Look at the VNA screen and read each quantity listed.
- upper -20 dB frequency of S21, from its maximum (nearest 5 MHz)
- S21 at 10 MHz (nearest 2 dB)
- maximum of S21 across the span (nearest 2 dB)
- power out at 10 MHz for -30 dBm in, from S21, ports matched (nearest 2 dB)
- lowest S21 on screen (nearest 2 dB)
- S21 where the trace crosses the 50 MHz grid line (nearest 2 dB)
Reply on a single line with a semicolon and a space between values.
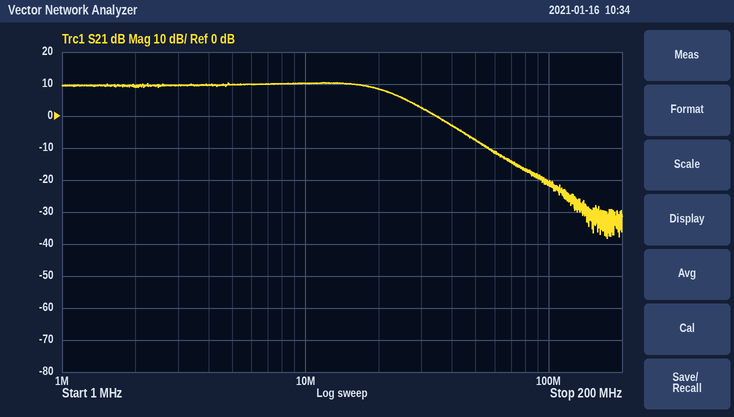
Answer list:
55 MHz; 10 dB; 10 dB; -20 dBm; -38 dB; -8 dB
